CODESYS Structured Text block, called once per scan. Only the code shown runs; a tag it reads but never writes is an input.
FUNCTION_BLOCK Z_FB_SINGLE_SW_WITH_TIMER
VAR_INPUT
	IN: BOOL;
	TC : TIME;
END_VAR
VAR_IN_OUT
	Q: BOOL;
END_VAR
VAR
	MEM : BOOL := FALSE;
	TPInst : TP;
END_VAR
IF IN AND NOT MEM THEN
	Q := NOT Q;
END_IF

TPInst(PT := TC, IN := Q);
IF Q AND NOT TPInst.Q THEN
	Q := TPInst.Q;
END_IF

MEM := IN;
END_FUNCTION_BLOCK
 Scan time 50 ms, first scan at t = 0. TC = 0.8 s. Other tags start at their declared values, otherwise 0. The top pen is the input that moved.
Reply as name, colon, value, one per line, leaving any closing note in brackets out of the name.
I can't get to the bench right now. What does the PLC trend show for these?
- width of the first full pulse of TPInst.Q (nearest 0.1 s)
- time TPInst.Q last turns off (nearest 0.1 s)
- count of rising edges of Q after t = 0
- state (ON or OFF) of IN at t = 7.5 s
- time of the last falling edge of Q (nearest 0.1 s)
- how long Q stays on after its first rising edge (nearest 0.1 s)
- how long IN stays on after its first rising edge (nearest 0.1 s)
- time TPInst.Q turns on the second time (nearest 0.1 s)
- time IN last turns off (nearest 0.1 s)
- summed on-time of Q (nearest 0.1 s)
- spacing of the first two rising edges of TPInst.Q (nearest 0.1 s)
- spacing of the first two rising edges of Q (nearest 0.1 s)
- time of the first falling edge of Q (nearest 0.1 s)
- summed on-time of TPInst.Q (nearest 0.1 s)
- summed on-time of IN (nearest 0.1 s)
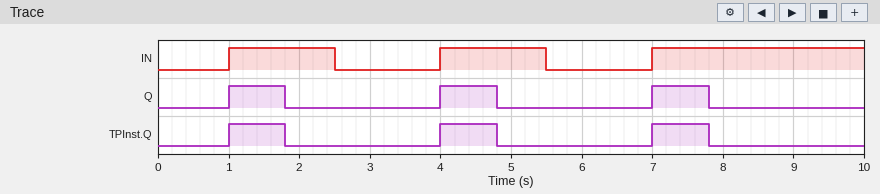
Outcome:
width of the first full pulse of TPInst.Q: 0.8 s
time TPInst.Q last turns off: 7.8 s
count of rising edges of Q after t = 0: 3
state (ON or OFF) of IN at t = 7.5 s: ON
time of the last falling edge of Q: 7.8 s
how long Q stays on after its first rising edge: 0.8 s
how long IN stays on after its first rising edge: 1.5 s
time TPInst.Q turns on the second time: 4.0 s
time IN last turns off: 5.5 s
summed on-time of Q: 2.4 s
spacing of the first two rising edges of TPInst.Q: 3.0 s
spacing of the first two rising edges of Q: 3.0 s
time of the first falling edge of Q: 1.8 s
summed on-time of TPInst.Q: 2.4 s
summed on-time of IN: 6.0 s
